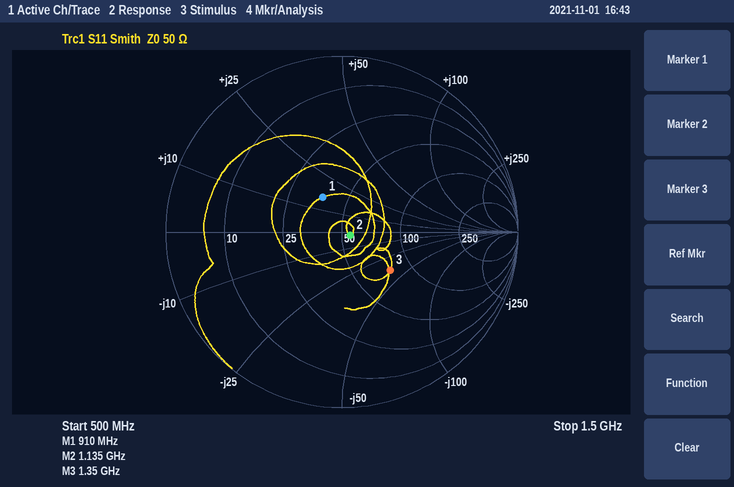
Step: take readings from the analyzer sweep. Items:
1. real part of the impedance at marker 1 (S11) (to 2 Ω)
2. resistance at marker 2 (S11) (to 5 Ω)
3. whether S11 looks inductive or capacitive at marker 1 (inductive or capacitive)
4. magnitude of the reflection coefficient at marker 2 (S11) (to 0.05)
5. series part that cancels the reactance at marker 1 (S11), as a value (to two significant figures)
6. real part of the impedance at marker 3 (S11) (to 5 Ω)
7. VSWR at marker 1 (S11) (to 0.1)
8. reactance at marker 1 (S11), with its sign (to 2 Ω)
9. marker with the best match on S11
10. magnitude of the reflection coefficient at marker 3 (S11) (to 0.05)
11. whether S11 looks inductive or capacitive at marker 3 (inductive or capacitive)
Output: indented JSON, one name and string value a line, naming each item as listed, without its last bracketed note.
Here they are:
{
  "real part of the impedance at marker 1 (S11)": "38 Ω",
  "resistance at marker 2 (S11)": "55 Ω",
  "whether S11 looks inductive or capacitive at marker 1": "inductive",
  "magnitude of the reflection coefficient at marker 2 (S11)": "0.05",
  "series part that cancels the reactance at marker 1 (S11), as a value": "11 pF",
  "real part of the impedance at marker 3 (S11)": "75 Ω",
  "VSWR at marker 1 (S11)": "1.6",
  "reactance at marker 1 (S11), with its sign": "+16 Ω",
  "marker with the best match on S11": "marker 2",
  "magnitude of the reflection coefficient at marker 3 (S11)": "0.35",
  "whether S11 looks inductive or capacitive at marker 3": "capacitive"
}
